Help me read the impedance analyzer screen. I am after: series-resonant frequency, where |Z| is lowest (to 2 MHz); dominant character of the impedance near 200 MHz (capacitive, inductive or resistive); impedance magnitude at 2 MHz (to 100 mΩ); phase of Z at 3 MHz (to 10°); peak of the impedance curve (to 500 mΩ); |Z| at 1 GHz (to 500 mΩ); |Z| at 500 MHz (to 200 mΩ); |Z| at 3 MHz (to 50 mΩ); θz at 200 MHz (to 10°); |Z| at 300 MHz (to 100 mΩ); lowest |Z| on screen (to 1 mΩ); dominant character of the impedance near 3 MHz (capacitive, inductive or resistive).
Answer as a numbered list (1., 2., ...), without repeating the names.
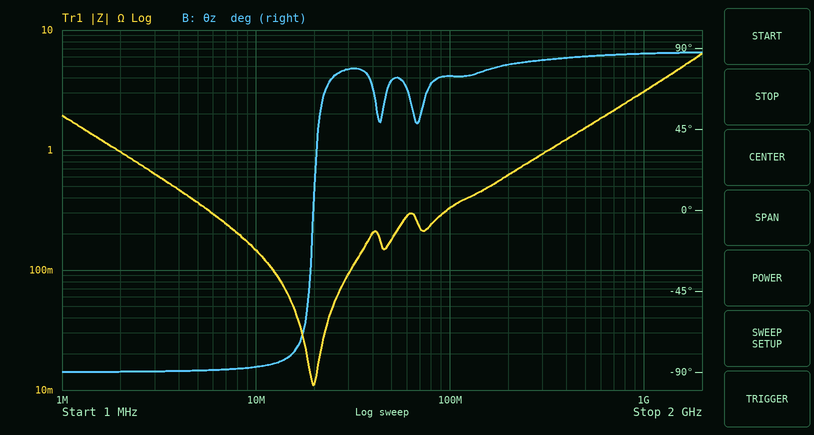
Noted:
1. 20 MHz
2. inductive
3. 1.0 Ω
4. -90°
5. 6.5 Ω
6. 3.0 Ω
7. 1.6 Ω
8. 650 mΩ
9. 80°
10. 900 mΩ
11. 11 mΩ
12. capacitive
